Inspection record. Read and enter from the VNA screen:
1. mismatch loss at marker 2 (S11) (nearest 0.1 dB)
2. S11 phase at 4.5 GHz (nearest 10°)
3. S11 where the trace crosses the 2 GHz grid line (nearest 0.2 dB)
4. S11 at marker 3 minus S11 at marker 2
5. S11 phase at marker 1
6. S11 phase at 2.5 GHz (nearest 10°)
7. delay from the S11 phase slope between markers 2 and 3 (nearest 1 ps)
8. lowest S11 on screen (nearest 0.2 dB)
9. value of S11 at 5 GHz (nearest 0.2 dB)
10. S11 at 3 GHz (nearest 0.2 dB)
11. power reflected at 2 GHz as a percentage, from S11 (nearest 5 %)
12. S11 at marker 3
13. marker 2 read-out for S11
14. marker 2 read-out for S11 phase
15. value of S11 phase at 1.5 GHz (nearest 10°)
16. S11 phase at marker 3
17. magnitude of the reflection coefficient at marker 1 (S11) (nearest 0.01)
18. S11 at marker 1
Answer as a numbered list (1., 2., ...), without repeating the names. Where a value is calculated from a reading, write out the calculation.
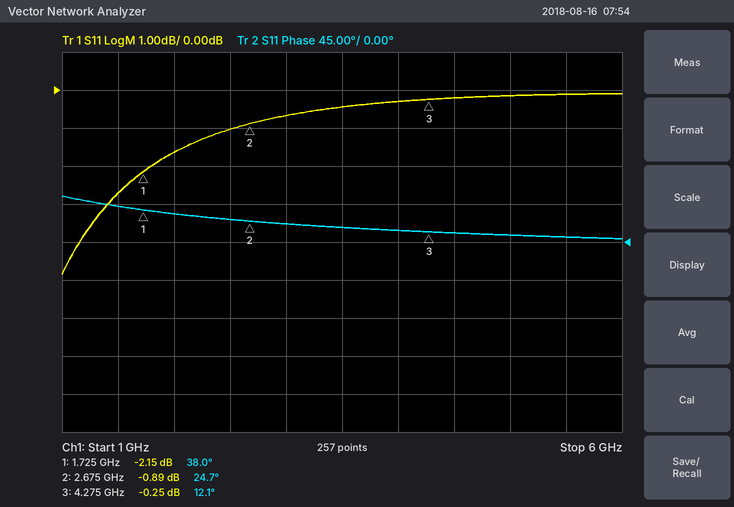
1. −10 log10(1 − 10^(-0.89/10)) ≈ 7.3 dB
2. 10°
3. -1.6 dB
4. -0.25 − (-0.89) = 0.64 dB
5. 38.0°
6. 30°
7. −(12.1° − (24.7°))/(360° × 1.6 GHz) ≈ 22 ps
8. -4.8 dB
9. -0.2 dB
10. -0.6 dB
11. 10^(-1.6/10) ≈ 69.2 %, so 70 % to the nearest 5 %
12. -0.25 dB
13. -0.89 dB
14. 24.7°
15. 40°
16. 12.1°
17. 10^(-2.15/20) ≈ 0.78
18. -2.15 dB
